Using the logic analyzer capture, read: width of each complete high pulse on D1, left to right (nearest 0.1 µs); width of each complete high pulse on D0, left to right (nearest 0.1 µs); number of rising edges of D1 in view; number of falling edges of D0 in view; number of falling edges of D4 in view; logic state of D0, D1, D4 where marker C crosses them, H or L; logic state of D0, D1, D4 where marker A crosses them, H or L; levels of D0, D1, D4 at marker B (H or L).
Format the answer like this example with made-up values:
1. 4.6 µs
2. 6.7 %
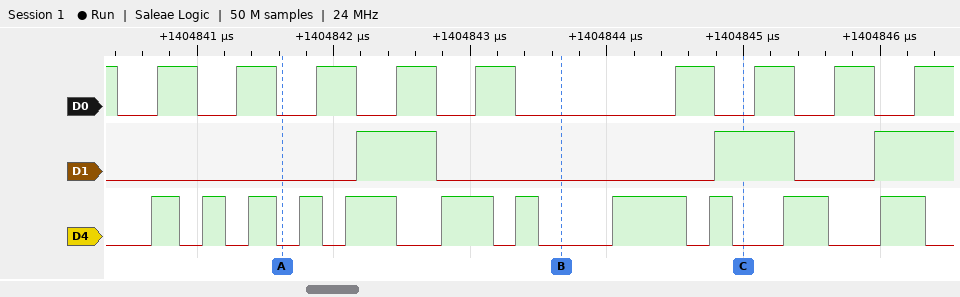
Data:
1. 0.6 µs, 0.6 µs
2. 0.3 µs, 0.3 µs, 0.3 µs, 0.3 µs, 0.3 µs, 0.3 µs, 0.3 µs, 0.3 µs
3. 3
4. 9
5. 11
6. D0=L, D1=H, D4=L
7. D0=L, D1=L, D4=L
8. D0=L, D1=L, D4=L
